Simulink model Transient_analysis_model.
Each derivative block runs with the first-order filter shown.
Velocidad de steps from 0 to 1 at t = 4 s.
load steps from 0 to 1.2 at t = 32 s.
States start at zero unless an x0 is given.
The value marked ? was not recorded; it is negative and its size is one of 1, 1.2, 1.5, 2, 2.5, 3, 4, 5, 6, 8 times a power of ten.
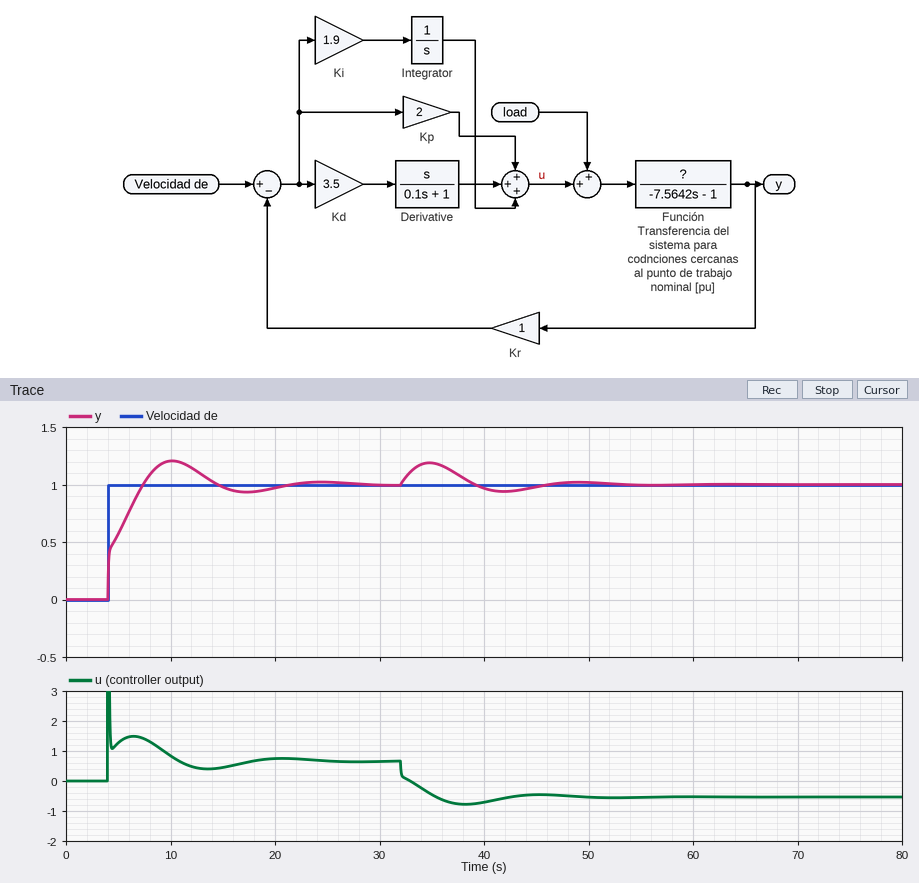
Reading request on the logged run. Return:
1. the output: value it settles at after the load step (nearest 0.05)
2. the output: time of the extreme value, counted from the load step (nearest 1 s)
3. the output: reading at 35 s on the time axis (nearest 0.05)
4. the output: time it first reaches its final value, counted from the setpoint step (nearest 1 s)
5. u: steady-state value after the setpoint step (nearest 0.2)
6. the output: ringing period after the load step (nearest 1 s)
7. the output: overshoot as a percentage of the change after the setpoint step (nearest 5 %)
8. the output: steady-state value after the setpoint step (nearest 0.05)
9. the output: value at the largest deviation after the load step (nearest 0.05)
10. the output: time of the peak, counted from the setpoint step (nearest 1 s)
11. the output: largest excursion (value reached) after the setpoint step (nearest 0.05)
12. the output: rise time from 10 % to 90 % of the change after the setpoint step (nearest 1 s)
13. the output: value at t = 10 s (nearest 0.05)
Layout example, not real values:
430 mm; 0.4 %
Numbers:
1.00; 3 s; 1.20; 3 s; 0.6; 14 s; 20 %; 1.00; 1.20; 6 s; 1.20; 3 s; 1.20
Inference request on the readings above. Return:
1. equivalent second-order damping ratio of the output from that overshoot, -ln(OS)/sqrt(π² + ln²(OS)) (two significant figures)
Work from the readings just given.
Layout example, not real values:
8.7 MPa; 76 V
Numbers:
0.46
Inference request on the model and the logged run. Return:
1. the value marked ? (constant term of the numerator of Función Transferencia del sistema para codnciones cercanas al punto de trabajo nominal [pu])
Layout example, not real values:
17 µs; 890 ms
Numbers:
-1.5
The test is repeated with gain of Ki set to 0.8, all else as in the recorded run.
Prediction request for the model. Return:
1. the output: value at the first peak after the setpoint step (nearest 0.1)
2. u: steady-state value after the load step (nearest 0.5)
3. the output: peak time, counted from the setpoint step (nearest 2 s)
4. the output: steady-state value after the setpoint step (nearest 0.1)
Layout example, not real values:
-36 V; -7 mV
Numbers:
1.1; -0.5; 10 s; 1.0
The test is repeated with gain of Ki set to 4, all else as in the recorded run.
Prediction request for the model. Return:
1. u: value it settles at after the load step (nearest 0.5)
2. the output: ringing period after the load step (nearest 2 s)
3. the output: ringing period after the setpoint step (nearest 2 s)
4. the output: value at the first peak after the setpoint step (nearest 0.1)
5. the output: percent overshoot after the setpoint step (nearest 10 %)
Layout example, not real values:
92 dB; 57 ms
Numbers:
-0.5; 10 s; 10 s; 1.3; 30 %
